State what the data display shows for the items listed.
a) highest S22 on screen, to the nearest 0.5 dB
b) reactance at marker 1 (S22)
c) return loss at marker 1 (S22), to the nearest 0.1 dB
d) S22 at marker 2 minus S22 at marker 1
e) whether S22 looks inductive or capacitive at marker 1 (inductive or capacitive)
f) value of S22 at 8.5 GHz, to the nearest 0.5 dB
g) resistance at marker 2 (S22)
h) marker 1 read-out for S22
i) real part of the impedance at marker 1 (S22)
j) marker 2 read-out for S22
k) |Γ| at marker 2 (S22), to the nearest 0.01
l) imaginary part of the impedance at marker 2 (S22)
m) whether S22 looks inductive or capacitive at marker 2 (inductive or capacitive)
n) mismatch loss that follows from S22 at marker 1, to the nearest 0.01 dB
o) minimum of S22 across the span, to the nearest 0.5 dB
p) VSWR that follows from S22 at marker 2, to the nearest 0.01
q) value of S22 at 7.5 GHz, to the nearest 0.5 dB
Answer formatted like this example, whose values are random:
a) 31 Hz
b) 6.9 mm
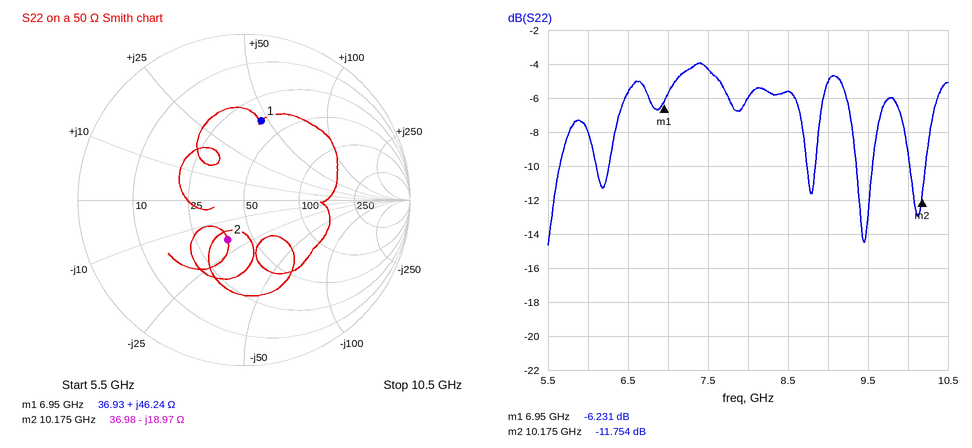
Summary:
a) -4.0 dB
b) +46.24 Ω
c) 6.2 dB
d) -5.523 dB
e) inductive
f) -5.5 dB
g) 36.98 Ω
h) -6.231 dB
i) 36.93 Ω
j) -11.754 dB
k) 0.26
l) -18.97 Ω
m) capacitive
n) 1.18 dB
o) -14.5 dB
p) 1.70
q) -4.5 dB
